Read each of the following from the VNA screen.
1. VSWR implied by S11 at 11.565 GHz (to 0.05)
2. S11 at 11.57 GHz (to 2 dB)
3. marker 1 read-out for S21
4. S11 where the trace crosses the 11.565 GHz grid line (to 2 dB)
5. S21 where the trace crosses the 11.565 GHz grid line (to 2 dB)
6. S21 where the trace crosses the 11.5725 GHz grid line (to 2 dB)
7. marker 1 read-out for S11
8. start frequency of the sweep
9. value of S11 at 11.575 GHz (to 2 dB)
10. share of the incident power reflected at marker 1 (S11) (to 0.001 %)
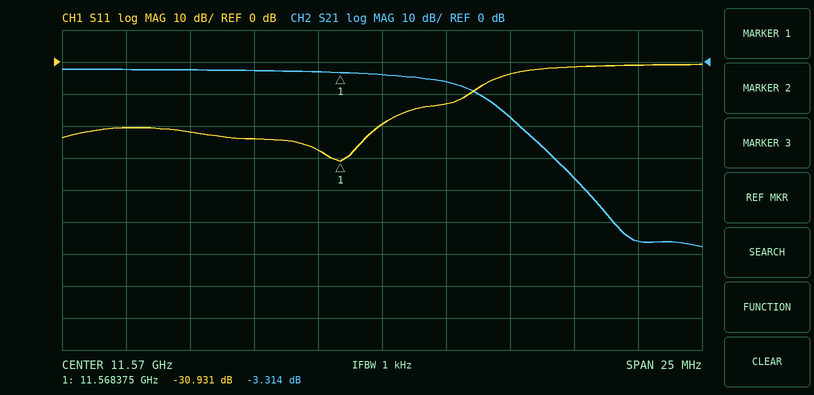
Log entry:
1.15
-20 dB
-3.314 dB
-24 dB
-2 dB
-6 dB
-30.931 dB
11.5575 GHz
-4 dB
0.081 %
